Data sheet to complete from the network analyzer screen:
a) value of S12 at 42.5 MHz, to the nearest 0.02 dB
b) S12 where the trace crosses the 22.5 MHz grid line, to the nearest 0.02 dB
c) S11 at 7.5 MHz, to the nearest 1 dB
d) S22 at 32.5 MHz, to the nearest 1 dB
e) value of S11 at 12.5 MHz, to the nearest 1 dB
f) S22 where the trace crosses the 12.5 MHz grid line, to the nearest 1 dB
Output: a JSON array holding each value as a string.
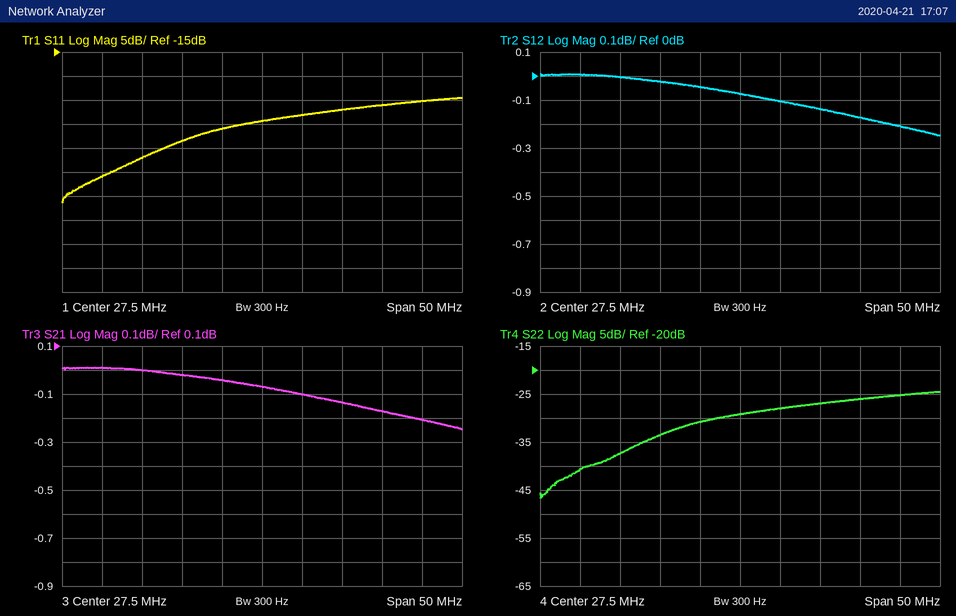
["-0.18 dB", "-0.04 dB", "-41 dB", "-28 dB", "-37 dB", "-37 dB"]
